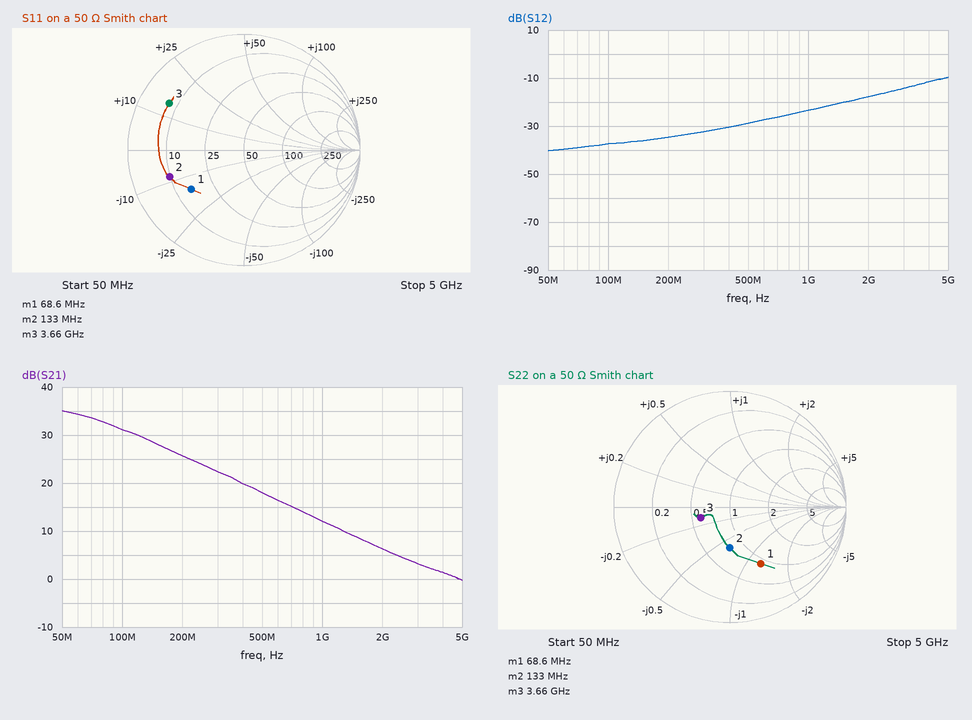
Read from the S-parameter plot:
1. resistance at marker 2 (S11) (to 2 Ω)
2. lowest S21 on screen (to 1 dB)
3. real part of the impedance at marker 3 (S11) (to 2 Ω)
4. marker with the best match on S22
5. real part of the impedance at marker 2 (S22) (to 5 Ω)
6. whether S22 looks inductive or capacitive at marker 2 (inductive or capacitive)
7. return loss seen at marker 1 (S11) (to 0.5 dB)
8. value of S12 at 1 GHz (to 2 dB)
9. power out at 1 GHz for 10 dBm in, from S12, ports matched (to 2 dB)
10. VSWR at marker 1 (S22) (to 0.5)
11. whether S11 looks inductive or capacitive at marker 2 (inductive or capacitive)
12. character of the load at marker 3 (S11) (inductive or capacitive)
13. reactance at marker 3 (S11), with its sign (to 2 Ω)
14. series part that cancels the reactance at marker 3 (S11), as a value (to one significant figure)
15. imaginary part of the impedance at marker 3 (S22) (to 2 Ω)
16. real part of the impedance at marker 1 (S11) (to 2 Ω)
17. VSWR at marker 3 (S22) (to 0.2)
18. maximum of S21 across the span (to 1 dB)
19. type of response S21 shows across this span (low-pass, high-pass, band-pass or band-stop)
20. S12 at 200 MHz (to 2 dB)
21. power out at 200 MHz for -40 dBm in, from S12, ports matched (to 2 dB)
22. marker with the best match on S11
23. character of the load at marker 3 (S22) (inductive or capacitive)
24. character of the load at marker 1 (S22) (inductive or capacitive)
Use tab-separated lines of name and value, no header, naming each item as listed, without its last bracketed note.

resistance at marker 2 (S11)	10 Ω
lowest S21 on screen	0 dB
real part of the impedance at marker 3 (S11)	8 Ω
marker with the best match on S22	marker 3
real part of the impedance at marker 2 (S22)	40 Ω
whether S22 looks inductive or capacitive at marker 2	capacitive
return loss seen at marker 1 (S11)	5.0 dB
value of S12 at 1 GHz	-24 dB
power out at 1 GHz for 10 dBm in, from S12, ports matched	-14 dBm
VSWR at marker 1 (S22)	3.5
whether S11 looks inductive or capacitive at marker 2	capacitive
character of the load at marker 3 (S11)	inductive
reactance at marker 3 (S11), with its sign	+14 Ω
series part that cancels the reactance at marker 3 (S11), as a value	3 pF
imaginary part of the impedance at marker 3 (S22)	-6 Ω
real part of the impedance at marker 1 (S11)	16 Ω
VSWR at marker 3 (S22)	1.8
maximum of S21 across the span	35 dB
type of response S21 shows across this span	low-pass
S12 at 200 MHz	-34 dB
power out at 200 MHz for -40 dBm in, from S12, ports matched	-74 dBm
marker with the best match on S11	marker 1
character of the load at marker 3 (S22)	capacitive
character of the load at marker 1 (S22)	capacitive
